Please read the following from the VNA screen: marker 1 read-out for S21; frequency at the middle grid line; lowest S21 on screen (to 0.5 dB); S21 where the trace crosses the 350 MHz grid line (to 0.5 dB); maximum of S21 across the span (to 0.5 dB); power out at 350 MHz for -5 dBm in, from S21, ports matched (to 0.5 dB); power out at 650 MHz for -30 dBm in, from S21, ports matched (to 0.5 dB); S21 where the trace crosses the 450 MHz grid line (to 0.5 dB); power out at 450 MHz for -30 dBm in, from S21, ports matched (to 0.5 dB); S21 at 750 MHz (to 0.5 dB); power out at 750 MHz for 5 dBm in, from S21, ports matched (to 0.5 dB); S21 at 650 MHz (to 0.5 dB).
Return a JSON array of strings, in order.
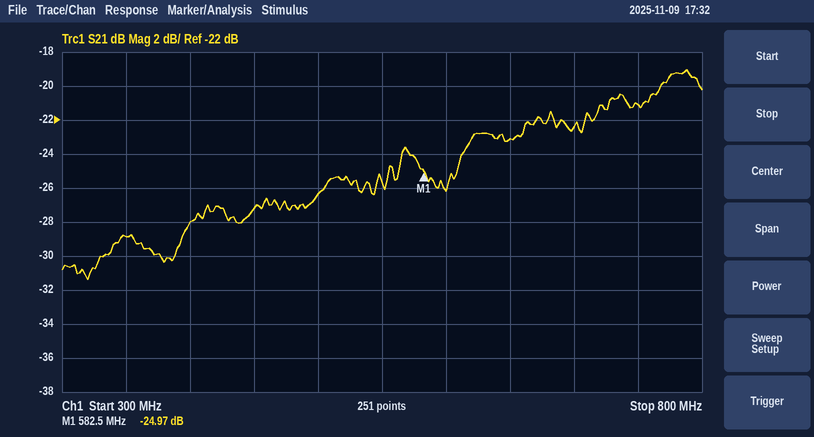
["-24.97 dB", "550 MHz", "-31.5 dB", "-29.0 dB", "-19.0 dB", "-34.0 dBm", "-53.0 dBm", "-27.0 dB", "-57.0 dBm", "-21.0 dB", "-16.0 dBm", "-23.0 dB"]
